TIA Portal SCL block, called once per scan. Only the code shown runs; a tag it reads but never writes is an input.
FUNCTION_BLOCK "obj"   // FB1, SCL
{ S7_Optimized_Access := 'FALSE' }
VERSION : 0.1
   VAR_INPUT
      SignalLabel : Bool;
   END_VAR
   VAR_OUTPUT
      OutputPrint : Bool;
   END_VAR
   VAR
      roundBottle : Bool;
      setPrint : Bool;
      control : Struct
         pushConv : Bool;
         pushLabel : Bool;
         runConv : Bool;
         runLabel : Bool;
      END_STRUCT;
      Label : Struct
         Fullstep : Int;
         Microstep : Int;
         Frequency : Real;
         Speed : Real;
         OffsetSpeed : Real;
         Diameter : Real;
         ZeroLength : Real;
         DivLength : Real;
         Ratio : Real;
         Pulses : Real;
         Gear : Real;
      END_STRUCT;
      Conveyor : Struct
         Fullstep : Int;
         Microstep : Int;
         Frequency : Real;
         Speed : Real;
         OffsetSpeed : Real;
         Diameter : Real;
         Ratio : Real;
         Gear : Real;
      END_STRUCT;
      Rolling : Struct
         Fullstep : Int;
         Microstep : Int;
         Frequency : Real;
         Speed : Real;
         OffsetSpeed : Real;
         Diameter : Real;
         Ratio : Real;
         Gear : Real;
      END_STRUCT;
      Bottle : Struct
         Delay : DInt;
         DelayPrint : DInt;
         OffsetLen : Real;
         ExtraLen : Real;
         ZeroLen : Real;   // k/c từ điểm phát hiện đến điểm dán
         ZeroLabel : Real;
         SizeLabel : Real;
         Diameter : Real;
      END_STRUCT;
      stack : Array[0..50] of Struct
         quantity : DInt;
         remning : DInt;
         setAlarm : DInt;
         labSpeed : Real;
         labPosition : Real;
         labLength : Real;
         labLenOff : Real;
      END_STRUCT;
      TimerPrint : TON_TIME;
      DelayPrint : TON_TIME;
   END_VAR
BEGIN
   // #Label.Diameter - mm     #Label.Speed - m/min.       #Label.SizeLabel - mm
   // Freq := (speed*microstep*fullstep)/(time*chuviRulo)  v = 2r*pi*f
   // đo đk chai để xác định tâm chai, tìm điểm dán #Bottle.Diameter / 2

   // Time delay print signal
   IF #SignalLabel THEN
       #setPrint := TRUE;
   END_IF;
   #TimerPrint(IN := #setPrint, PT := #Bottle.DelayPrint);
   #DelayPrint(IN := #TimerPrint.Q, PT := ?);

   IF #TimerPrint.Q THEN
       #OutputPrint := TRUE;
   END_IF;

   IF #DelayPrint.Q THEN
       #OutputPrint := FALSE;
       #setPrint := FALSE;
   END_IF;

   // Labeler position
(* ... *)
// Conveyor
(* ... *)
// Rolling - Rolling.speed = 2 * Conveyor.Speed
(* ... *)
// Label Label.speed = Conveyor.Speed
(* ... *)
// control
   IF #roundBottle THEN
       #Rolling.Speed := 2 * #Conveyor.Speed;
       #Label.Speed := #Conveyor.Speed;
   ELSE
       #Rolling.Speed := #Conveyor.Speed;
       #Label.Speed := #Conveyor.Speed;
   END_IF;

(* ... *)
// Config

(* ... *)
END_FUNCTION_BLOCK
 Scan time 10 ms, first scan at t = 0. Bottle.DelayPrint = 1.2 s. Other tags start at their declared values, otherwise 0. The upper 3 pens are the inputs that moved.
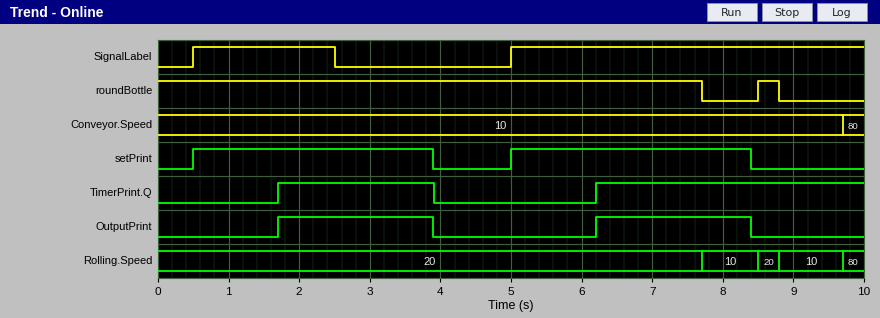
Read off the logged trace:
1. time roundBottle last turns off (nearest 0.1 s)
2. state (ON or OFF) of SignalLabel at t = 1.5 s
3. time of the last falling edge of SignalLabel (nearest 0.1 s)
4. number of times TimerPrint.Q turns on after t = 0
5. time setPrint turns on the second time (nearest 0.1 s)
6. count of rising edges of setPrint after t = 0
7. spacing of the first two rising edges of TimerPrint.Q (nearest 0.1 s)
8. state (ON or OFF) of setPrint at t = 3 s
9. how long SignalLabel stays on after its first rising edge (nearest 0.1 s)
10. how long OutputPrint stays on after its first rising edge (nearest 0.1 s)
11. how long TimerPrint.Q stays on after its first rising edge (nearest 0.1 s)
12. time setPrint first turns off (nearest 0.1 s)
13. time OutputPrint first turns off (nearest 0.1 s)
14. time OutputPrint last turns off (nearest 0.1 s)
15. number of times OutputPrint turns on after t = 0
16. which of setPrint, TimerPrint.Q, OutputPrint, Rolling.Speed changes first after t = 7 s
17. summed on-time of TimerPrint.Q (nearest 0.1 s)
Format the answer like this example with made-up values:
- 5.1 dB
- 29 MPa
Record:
- 8.8 s
- ON
- 2.5 s
- 2
- 5.0 s
- 2
- 4.5 s
- ON
- 2.0 s
- 2.2 s
- 2.2 s
- 3.9 s
- 3.9 s
- 8.4 s
- 2
- Rolling.Speed
- 6.0 s
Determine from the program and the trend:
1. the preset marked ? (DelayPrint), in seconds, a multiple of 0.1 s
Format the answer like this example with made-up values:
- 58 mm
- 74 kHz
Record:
- 2.2 s
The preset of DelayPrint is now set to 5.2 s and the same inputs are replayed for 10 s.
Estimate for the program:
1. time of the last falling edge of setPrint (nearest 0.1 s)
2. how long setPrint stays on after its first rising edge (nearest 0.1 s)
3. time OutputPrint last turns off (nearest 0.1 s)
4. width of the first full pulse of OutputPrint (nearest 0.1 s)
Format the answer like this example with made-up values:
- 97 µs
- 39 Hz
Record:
- 6.9 s
- 6.4 s
- 6.9 s
- 5.2 s
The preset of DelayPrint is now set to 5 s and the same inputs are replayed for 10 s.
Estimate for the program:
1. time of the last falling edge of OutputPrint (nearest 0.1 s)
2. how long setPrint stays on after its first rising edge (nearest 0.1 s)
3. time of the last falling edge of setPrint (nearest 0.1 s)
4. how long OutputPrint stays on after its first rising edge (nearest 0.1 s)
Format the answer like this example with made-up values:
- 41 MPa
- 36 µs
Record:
- 6.7 s
- 6.2 s
- 6.7 s
- 5.0 s
